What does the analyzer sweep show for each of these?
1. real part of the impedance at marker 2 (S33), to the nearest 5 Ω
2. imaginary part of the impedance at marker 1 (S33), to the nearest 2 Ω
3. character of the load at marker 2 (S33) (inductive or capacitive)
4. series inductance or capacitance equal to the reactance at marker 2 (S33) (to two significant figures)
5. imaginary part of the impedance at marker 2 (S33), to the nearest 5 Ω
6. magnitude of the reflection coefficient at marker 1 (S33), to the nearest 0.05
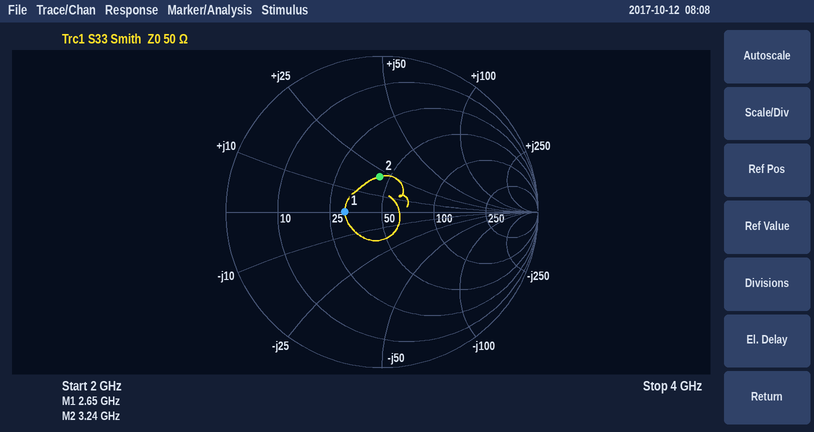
45 Ω
0 Ω
inductive
1.0 nH
+20 Ω
0.25
